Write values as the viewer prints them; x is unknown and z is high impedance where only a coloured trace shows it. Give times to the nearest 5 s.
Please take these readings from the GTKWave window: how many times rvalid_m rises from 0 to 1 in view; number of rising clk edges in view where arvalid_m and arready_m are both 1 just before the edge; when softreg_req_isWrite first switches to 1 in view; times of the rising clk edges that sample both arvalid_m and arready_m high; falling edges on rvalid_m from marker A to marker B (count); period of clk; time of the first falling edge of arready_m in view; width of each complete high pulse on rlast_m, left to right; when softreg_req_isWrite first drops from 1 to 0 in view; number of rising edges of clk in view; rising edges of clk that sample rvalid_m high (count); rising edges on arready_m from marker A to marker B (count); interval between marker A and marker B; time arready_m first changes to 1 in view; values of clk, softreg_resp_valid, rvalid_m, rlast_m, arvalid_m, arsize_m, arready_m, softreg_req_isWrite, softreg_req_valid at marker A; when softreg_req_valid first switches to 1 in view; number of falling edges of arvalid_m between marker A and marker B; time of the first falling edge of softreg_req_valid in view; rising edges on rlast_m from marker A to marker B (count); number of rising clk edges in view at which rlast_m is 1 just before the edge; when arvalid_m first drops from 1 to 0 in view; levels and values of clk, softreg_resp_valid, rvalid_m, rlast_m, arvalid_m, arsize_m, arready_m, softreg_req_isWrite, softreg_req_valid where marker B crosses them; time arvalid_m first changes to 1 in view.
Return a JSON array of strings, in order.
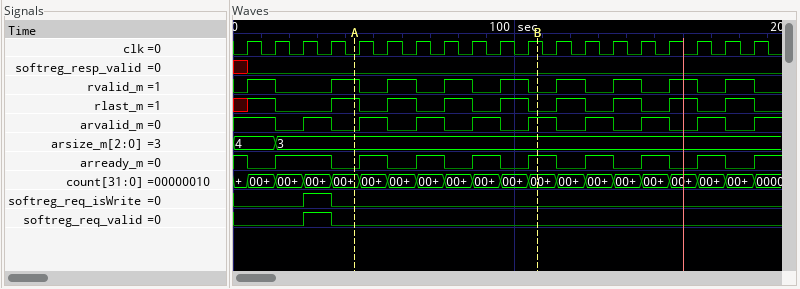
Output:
["9", "9", "25 s", "5 s, 35 s, 55 s, 75 s, 95 s, 115 s, 135 s, 155 s, 175 s", "4", "10 s", "5 s", "10 s, 10 s, 10 s, 10 s, 10 s, 10 s, 10 s, 10 s", "35 s", "19", "9", "4", "65 s", "15 s", "clk=0, softreg_resp_valid=0, rvalid_m=1, rlast_m=1, arvalid_m=0, arsize_m=3, arready_m=0, softreg_req_isWrite=0, softreg_req_valid=0", "25 s", "3", "35 s", "3", "9", "15 s", "clk=1, softreg_resp_valid=0, rvalid_m=0, rlast_m=0, arvalid_m=1, arsize_m=3, arready_m=1, softreg_req_isWrite=0, softreg_req_valid=0", "25 s"]
